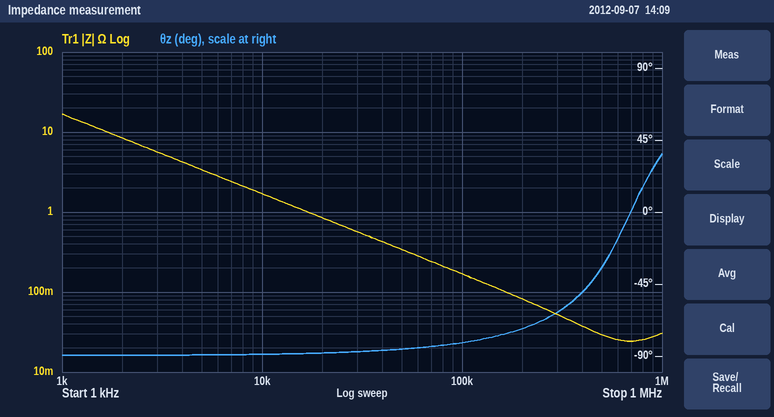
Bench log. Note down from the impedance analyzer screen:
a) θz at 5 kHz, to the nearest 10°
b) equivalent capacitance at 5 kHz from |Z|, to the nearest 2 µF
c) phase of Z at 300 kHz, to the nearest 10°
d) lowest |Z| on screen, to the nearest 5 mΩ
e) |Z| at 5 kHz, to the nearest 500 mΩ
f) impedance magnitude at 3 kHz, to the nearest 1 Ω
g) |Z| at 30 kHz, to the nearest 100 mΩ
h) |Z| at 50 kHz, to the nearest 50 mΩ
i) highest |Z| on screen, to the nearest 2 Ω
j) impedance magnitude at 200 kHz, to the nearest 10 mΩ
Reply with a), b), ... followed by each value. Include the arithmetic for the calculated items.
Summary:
a) -90°
b) C = 1/(2π × 5 kHz × 3.5 Ω) ≈ 9.09 µF, so 10 µF to the nearest 2 µF
c) -60°
d) 25 mΩ
e) 3.5 Ω
f) 6 Ω
g) 600 mΩ
h) 350 mΩ
i) 16 Ω
j) 80 mΩ
